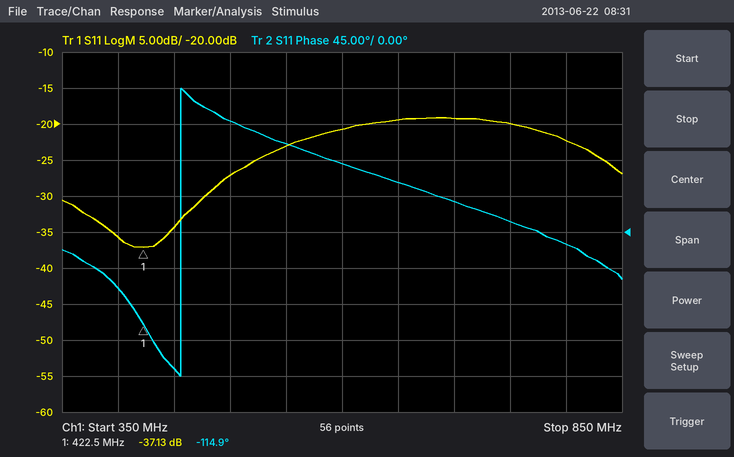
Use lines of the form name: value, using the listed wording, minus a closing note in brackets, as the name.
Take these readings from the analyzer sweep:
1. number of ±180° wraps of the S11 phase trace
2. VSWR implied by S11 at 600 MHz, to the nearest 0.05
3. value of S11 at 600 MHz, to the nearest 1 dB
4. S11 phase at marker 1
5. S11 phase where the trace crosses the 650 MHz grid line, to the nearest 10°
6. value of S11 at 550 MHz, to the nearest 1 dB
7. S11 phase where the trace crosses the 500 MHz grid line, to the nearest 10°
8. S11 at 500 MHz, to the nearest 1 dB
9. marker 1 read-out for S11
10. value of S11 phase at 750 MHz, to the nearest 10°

number of ±180° wraps of the S11 phase trace: 1
VSWR implied by S11 at 600 MHz, to the nearest 0.05: 1.20
value of S11 at 600 MHz, to the nearest 1 dB: -21 dB
S11 phase at marker 1: -114.9°
S11 phase where the trace crosses the 650 MHz grid line, to the nearest 10°: 60°
value of S11 at 550 MHz, to the nearest 1 dB: -23 dB
S11 phase where the trace crosses the 500 MHz grid line, to the nearest 10°: 140°
S11 at 500 MHz, to the nearest 1 dB: -27 dB
marker 1 read-out for S11: -37.13 dB
value of S11 phase at 750 MHz, to the nearest 10°: 10°
